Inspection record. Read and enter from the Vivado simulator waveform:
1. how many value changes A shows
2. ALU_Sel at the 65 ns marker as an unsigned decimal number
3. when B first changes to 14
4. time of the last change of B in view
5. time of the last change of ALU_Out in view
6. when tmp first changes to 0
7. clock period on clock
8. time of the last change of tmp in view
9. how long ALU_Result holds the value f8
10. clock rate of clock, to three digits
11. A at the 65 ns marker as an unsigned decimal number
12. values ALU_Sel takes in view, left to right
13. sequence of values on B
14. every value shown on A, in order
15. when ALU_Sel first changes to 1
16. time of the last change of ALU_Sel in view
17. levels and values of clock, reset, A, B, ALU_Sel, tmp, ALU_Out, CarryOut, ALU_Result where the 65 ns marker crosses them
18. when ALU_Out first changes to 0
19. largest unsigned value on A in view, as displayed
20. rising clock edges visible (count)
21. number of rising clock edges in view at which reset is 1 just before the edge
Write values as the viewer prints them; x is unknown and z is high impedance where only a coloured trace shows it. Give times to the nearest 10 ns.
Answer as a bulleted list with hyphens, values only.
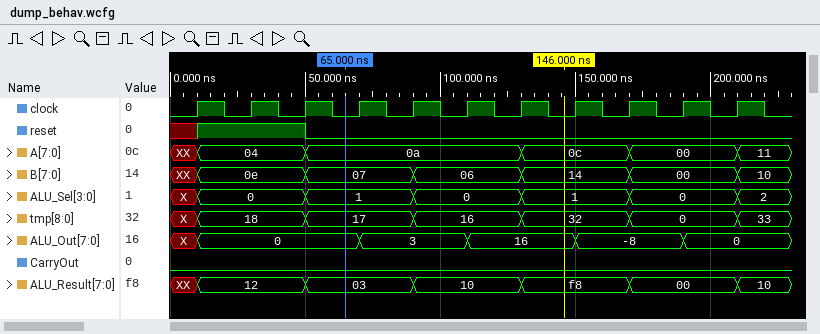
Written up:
- 5
- 1
- 130 ns
- 210 ns
- 190 ns
- 170 ns
- 20 ns
- 210 ns
- 40 ns
- 50.0 MHz
- 10
- X, 0, 1, 0, 1, 0, 2
- XX, 0e, 07, 06, 14, 00, 10
- XX, 04, 0a, 0c, 00, 11
- 50 ns
- 210 ns
- clock=0, reset=0, A=0a, B=07, ALU_Sel=1, tmp=17, ALU_Out=0, CarryOut=0, ALU_Result=03
- 10 ns
- 11
- 11
- 2
